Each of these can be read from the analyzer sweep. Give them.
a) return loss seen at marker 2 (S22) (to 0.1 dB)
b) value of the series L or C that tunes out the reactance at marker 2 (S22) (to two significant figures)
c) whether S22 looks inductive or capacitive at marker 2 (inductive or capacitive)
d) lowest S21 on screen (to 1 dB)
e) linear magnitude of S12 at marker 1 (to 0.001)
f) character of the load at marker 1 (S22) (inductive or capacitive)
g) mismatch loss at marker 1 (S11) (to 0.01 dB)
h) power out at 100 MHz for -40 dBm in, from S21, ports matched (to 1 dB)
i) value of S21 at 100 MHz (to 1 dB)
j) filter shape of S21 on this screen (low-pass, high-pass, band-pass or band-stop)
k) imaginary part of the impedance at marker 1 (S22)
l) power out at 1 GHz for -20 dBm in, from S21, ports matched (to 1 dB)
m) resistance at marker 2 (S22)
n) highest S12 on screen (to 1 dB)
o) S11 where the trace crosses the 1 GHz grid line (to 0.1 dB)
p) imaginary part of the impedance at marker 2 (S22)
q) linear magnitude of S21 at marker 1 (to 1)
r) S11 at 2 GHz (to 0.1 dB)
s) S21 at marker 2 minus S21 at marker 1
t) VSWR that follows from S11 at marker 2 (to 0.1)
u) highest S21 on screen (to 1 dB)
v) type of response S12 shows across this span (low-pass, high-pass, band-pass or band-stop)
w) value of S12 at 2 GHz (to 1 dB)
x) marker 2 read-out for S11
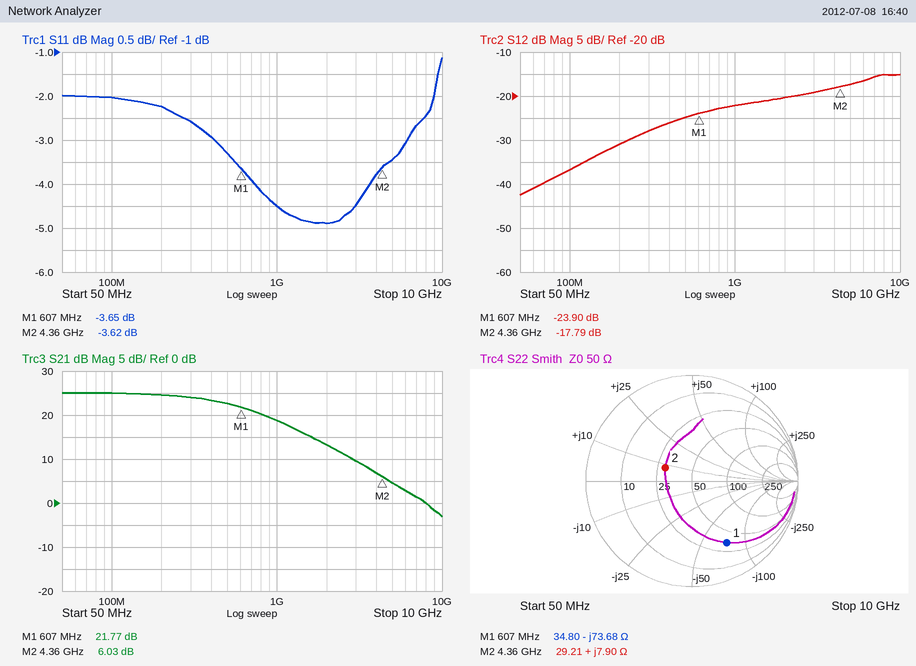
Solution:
11.1 dB
4.6 pF
inductive
-3 dB
0.064
capacitive
2.45 dB
-15 dBm
25 dB
low-pass
-73.68 Ω
-1 dBm
29.21 Ω
-15 dB
-4.5 dB
+7.90 Ω
12
-4.9 dB
-15.74 dB
4.9
25 dB
high-pass
-20 dB
-3.62 dB
